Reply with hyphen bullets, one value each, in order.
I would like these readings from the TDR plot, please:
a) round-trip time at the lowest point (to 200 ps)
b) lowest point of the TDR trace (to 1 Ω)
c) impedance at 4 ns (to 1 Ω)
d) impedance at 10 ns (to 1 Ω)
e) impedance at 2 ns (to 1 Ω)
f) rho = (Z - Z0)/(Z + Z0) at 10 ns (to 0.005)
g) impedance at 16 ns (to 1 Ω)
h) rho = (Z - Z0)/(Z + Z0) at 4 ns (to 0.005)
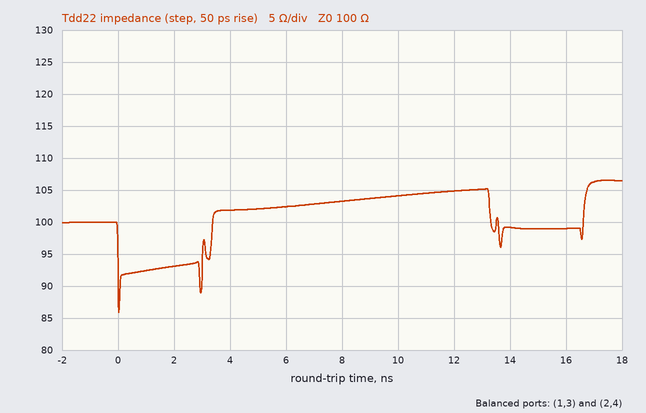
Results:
- 0.0 ns
- 86 Ω
- 102 Ω
- 104 Ω
- 93 Ω
- +0.020
- 99 Ω
- +0.010
